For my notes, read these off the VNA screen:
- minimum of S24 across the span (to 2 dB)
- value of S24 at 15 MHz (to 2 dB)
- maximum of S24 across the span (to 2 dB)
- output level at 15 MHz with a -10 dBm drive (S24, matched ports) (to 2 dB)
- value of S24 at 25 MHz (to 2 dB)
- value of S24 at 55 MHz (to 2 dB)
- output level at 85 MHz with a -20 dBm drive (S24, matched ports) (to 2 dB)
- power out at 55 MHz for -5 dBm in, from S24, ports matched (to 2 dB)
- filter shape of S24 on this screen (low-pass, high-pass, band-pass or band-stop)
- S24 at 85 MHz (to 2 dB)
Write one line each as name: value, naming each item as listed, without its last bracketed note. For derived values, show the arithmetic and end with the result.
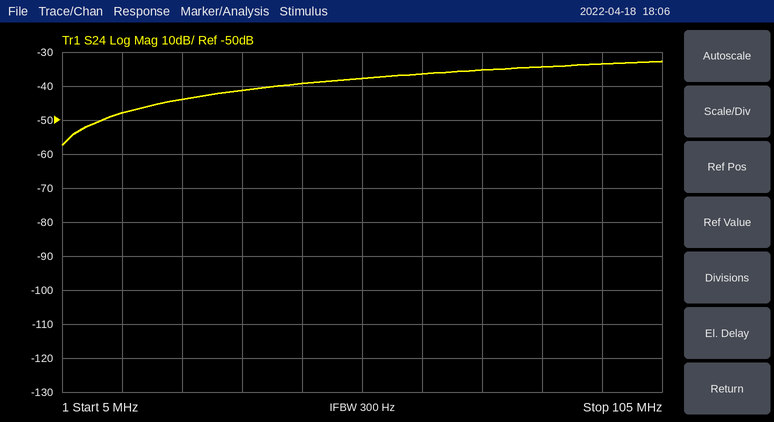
minimum of S24 across the span: -58 dB
value of S24 at 15 MHz: -48 dB
maximum of S24 across the span: -32 dB
output level at 15 MHz with a -10 dBm drive (S24, matched ports): -10 dBm + (-48 dB) = -58 dBm
value of S24 at 25 MHz: -44 dB
value of S24 at 55 MHz: -38 dB
output level at 85 MHz with a -20 dBm drive (S24, matched ports): -20 dBm + (-34 dB) = -54 dBm
power out at 55 MHz for -5 dBm in, from S24, ports matched: -5 dBm + (-38 dB) = -42 dBm
filter shape of S24 on this screen: high-pass
S24 at 85 MHz: -34 dB
